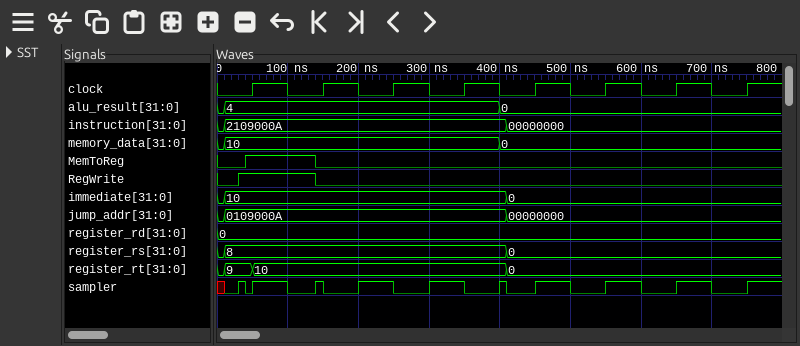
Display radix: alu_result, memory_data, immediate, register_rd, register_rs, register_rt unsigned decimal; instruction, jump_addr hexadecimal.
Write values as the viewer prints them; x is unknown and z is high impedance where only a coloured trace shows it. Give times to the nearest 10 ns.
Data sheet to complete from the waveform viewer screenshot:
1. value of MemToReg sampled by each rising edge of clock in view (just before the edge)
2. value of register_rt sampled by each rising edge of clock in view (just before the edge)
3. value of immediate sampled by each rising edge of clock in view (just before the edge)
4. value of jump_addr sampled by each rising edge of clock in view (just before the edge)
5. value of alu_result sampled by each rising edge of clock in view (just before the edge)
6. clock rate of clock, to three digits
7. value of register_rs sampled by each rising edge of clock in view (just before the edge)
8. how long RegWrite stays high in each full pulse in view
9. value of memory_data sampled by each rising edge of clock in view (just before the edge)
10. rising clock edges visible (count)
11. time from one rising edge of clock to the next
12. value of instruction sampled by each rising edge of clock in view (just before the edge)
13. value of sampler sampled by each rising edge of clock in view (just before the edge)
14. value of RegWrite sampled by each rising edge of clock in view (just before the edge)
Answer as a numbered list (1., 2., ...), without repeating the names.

1. 1 0 0 0 0 0 0 0
2. 9, 10, 10, 10, 0, 0, 0, 0
3. 10, 10, 10, 10, 0, 0, 0, 0
4. 0109000A, 0109000A, 0109000A, 0109000A, 00000000, 00000000, 00000000, 00000000
5. 4, 4, 4, 4, 0, 0, 0, 0
6. 10.0 MHz
7. 8, 8, 8, 8, 0, 0, 0, 0
8. 110 ns
9. 10, 10, 10, 10, 0, 0, 0, 0
10. 8
11. 100 ns
12. 2109000A, 2109000A, 2109000A, 2109000A, 00000000, 00000000, 00000000, 00000000
13. 0 1 1 1 0 0 0 0
14. 1 0 0 0 0 0 0 0
